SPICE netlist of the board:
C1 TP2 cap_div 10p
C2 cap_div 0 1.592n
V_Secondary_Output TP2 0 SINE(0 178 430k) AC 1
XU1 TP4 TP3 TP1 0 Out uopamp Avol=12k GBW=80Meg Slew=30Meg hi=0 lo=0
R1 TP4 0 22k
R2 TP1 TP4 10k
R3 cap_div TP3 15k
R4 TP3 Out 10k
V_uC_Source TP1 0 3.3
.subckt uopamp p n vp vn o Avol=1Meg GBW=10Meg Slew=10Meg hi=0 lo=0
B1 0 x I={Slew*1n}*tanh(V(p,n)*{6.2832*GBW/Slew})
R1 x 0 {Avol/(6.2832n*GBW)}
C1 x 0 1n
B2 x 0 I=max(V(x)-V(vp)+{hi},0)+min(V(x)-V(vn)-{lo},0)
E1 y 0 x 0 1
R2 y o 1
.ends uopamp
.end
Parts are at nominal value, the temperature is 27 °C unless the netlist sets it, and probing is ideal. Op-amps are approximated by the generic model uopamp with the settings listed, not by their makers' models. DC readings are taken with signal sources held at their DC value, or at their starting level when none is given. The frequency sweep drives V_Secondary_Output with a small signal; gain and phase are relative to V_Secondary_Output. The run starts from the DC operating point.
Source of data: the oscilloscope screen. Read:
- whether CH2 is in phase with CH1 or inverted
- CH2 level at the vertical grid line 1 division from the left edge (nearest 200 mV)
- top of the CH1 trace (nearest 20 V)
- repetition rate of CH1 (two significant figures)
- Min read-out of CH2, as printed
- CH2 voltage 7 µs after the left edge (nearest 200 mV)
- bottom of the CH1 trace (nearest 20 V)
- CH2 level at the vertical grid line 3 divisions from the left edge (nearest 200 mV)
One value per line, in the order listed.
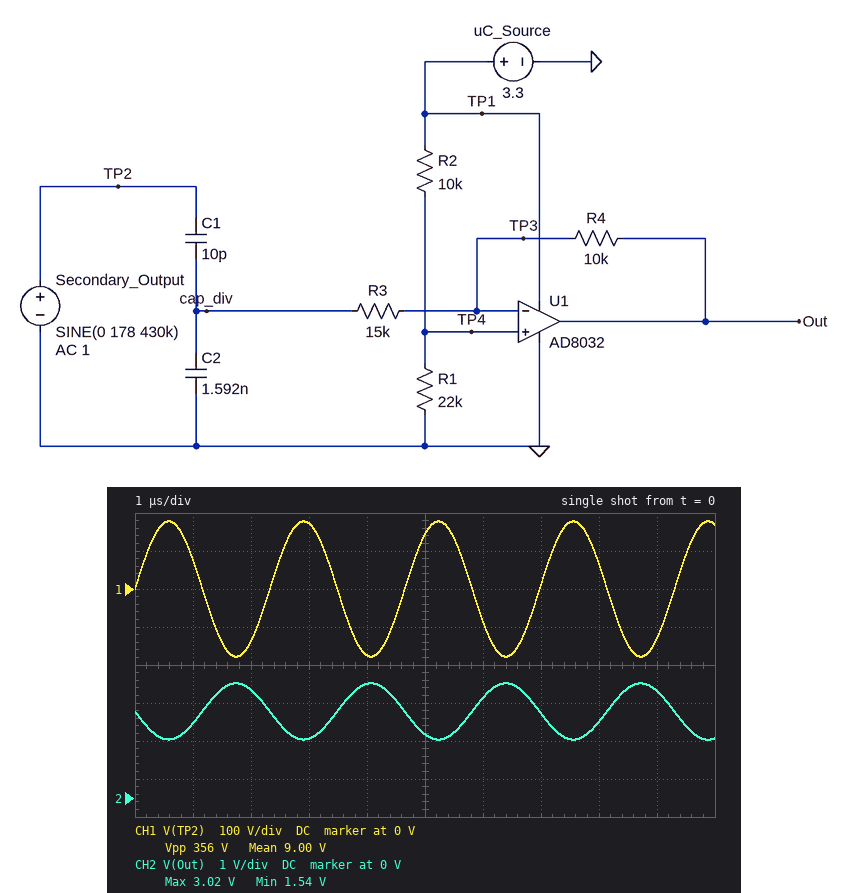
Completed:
inverted
2.0 V
180 V
430 kHz
1.54 V
2.2 V
-180 V
1.6 V
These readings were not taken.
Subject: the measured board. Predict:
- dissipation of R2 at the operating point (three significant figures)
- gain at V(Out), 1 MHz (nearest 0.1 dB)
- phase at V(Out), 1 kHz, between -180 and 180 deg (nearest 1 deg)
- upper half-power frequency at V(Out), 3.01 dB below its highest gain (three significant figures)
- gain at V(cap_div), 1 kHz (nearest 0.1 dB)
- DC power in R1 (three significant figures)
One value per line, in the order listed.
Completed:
106 µW
-47.6 dB
-99 deg
48.0 MHz
-60.6 dB
234 µW
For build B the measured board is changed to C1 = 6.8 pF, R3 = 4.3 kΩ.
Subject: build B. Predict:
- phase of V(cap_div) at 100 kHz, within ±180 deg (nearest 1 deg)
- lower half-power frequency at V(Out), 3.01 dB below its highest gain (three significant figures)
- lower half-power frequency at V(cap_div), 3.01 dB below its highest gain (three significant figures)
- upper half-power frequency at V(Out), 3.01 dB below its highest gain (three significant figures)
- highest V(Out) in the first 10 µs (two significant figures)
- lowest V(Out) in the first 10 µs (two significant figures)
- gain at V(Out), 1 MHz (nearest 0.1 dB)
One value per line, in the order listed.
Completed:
13 deg
23.1 kHz
23.2 kHz
24.1 MHz
3.3 V
600 mV
-40.1 dB
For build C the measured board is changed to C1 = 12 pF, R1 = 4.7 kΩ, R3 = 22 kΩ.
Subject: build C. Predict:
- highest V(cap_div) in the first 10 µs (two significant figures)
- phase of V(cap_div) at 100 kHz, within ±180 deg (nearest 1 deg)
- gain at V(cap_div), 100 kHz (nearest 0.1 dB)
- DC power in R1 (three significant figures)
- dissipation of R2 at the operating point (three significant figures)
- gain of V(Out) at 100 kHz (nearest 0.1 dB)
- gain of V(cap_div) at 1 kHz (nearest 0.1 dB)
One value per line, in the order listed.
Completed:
2.4 V
3 deg
-42.5 dB
237 µW
504 µW
-49.4 dB
-55.8 dB
